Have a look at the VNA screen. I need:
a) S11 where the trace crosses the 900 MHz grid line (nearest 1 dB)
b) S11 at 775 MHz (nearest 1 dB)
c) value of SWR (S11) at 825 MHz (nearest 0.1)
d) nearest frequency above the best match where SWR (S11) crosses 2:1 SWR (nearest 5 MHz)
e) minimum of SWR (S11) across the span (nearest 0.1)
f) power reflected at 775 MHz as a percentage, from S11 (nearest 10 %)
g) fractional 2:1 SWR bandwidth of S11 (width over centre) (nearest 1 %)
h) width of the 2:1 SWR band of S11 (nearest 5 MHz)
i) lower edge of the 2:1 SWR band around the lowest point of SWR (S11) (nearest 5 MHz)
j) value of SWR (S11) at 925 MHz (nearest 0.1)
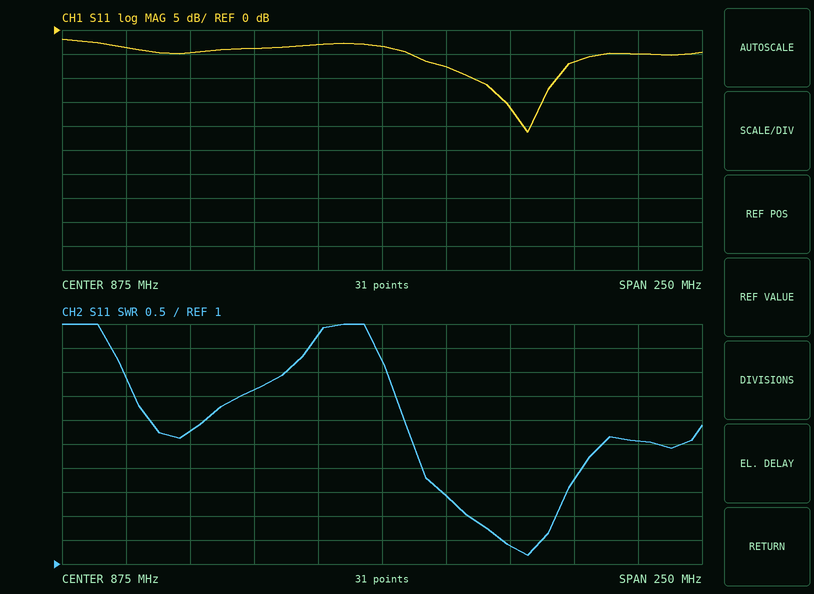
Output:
-8 dB
-4 dB
4.6
945 MHz
1.2
40 %
4 %
35 MHz
910 MHz
1.4
